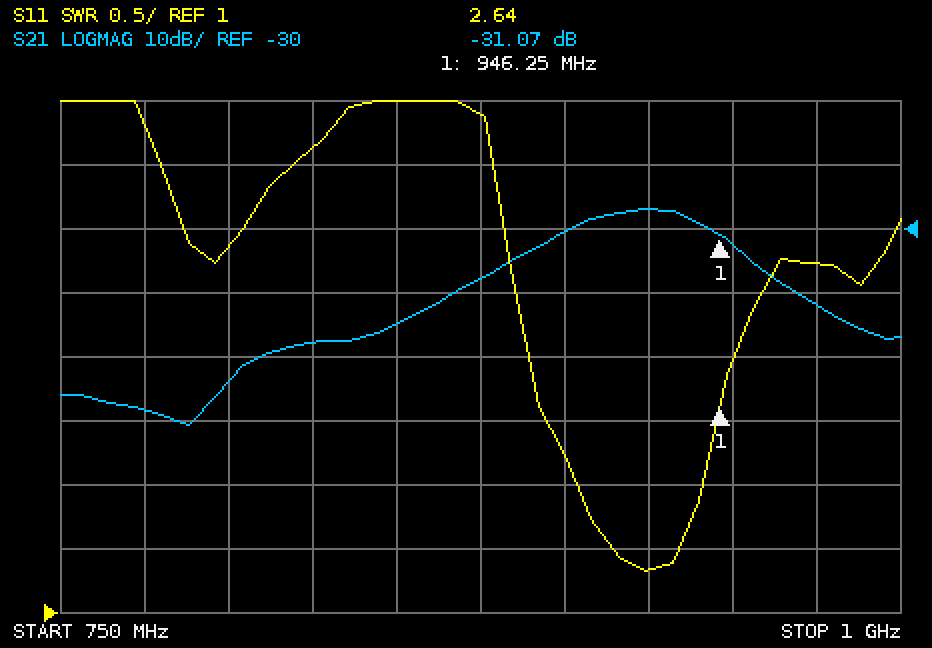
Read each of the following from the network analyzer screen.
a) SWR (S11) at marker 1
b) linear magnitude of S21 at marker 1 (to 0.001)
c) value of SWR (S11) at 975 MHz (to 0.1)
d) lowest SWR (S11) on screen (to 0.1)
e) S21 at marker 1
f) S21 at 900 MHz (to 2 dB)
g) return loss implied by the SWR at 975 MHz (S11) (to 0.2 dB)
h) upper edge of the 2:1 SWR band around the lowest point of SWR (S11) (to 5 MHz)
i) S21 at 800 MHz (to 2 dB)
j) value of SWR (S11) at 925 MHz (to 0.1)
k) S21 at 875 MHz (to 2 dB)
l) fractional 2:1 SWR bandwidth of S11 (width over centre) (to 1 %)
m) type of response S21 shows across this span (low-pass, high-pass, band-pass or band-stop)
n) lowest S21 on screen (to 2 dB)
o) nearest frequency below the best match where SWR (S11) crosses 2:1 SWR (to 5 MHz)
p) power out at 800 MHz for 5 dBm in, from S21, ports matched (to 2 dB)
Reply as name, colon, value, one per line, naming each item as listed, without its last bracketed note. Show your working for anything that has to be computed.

SWR (S11) at marker 1: 2.64
linear magnitude of S21 at marker 1: 10^(-31.07/20) ≈ 0.028
value of SWR (S11) at 975 MHz: 3.7
lowest SWR (S11) on screen: 1.3
S21 at marker 1: -31.07 dB
S21 at 900 MHz: -30 dB
return loss implied by the SWR at 975 MHz (S11): −20 log10((3.7 − 1)/(3.7 + 1)) ≈ 4.8 dB
upper edge of the 2:1 SWR band around the lowest point of SWR (S11): 940 MHz
S21 at 800 MHz: -54 dB
value of SWR (S11) at 925 MHz: 1.3
S21 at 875 MHz: -38 dB
fractional 2:1 SWR bandwidth of S11 (width over centre): 35 MHz / 922.5 MHz ≈ 4 %
type of response S21 shows across this span: band-pass
lowest S21 on screen: -60 dB
nearest frequency below the best match where SWR (S11) crosses 2:1 SWR: 905 MHz
power out at 800 MHz for 5 dBm in, from S21, ports matched: 5 dBm + (-54 dB) = -48 dBm
